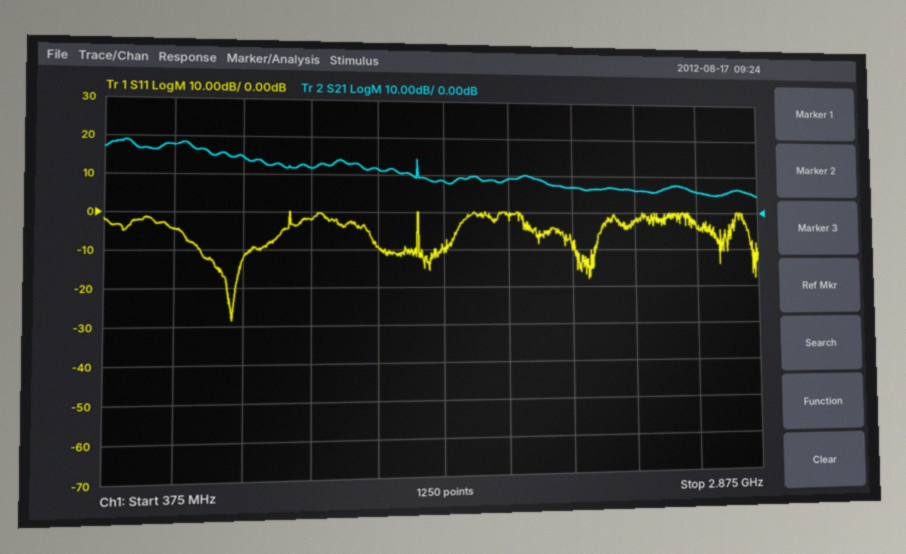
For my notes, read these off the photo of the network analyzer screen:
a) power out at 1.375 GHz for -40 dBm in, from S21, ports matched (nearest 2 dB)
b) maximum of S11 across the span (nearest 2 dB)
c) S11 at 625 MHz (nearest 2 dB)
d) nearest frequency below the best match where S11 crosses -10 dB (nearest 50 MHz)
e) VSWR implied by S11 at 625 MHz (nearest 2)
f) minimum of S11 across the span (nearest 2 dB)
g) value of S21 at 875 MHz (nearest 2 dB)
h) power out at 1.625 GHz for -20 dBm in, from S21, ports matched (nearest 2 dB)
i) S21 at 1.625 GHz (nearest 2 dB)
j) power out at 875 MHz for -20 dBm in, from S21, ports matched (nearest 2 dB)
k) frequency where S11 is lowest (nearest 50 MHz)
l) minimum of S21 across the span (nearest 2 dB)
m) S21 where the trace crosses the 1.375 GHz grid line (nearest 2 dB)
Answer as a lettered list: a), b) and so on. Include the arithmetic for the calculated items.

a) -40 dBm + (12 dB) = -28 dBm
b) 0 dB
c) -4 dB
d) 700 MHz
e) |Γ| = 10^(-4/20) = 0.6310; VSWR = (1 + 0.6310)/(1 − 0.6310) ≈ 4
f) -28 dB
g) 14 dB
h) -20 dBm + (8 dB) = -12 dBm
i) 8 dB
j) -20 dBm + (14 dB) = -6 dBm
k) 850 MHz
l) 4 dB
m) 12 dB
